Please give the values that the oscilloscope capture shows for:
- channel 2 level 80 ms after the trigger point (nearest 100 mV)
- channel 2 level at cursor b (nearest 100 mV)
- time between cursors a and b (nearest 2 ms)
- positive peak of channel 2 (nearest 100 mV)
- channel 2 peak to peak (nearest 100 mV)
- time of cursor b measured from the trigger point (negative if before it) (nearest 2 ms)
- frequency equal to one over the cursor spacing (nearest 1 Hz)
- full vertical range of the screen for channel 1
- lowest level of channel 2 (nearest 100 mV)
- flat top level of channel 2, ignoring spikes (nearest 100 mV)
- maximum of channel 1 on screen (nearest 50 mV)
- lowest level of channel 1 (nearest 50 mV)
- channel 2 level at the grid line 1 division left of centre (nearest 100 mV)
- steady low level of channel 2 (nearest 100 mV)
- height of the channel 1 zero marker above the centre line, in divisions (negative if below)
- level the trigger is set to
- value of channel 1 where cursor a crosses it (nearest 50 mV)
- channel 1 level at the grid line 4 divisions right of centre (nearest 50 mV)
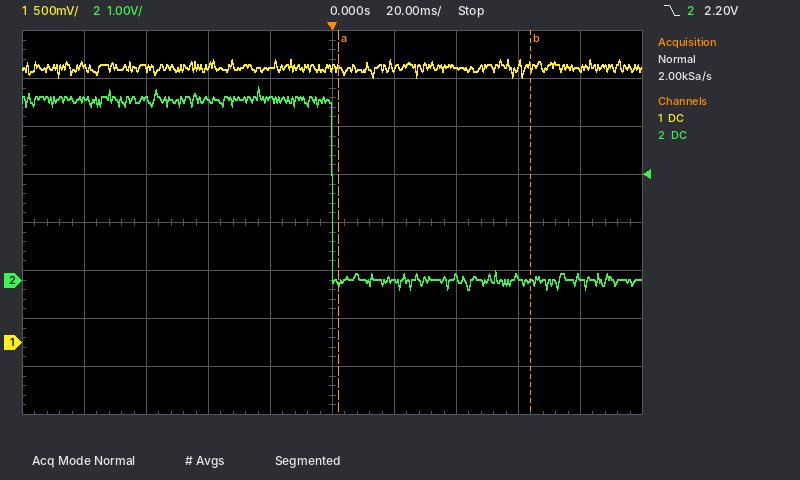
100 mV
0.0 V
62 ms
4.0 V
4.2 V
+64 ms
16 Hz
4 V
-200 mV
3.8 V
2.95 V
2.75 V
3.8 V
0.0 V
-2.5 div
2.20 V
2.85 V
2.85 V
